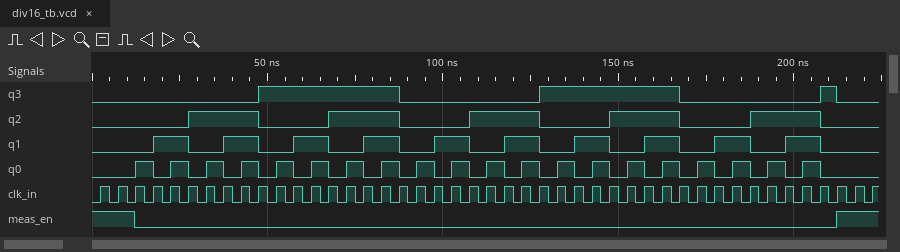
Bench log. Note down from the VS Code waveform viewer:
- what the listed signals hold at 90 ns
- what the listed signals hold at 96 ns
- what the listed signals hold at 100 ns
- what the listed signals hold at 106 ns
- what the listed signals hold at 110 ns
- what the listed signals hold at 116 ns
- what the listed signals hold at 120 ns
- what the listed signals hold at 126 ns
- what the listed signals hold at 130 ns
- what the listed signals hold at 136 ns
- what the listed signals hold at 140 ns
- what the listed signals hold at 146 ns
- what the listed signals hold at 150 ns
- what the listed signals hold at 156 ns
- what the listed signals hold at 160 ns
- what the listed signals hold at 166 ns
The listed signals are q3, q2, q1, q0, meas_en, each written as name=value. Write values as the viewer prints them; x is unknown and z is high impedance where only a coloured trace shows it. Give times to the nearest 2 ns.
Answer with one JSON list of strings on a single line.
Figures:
["q3=0, q2=0, q1=0, q0=0, meas_en=0", "q3=0, q2=0, q1=0, q0=1, meas_en=0", "q3=0, q2=0, q1=1, q0=0, meas_en=0", "q3=0, q2=0, q1=1, q0=1, meas_en=0", "q3=0, q2=1, q1=0, q0=0, meas_en=0", "q3=0, q2=1, q1=0, q0=1, meas_en=0", "q3=0, q2=1, q1=1, q0=0, meas_en=0", "q3=0, q2=1, q1=1, q0=1, meas_en=0", "q3=1, q2=0, q1=0, q0=0, meas_en=0", "q3=1, q2=0, q1=0, q0=1, meas_en=0", "q3=1, q2=0, q1=1, q0=0, meas_en=0", "q3=1, q2=0, q1=1, q0=1, meas_en=0", "q3=1, q2=1, q1=0, q0=0, meas_en=0", "q3=1, q2=1, q1=0, q0=1, meas_en=0", "q3=1, q2=1, q1=1, q0=0, meas_en=0", "q3=1, q2=1, q1=1, q0=1, meas_en=0"]
